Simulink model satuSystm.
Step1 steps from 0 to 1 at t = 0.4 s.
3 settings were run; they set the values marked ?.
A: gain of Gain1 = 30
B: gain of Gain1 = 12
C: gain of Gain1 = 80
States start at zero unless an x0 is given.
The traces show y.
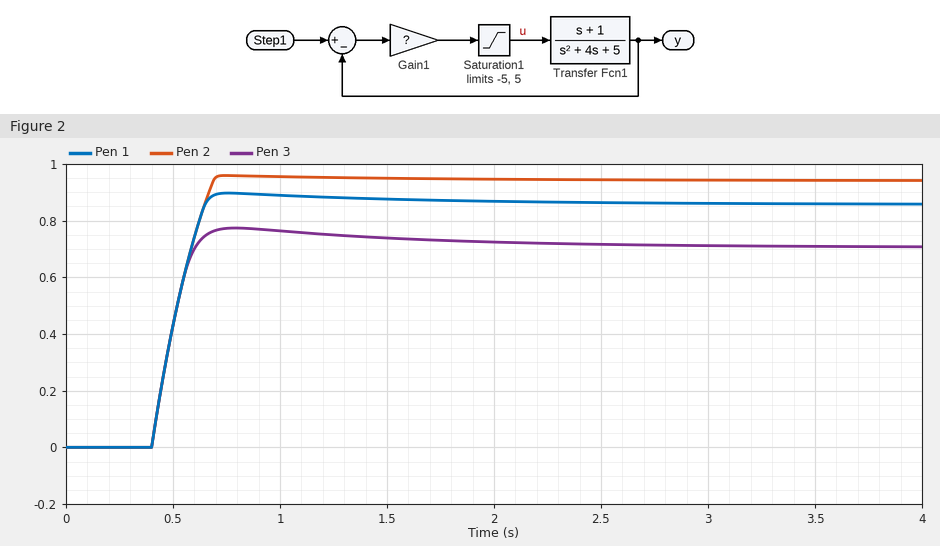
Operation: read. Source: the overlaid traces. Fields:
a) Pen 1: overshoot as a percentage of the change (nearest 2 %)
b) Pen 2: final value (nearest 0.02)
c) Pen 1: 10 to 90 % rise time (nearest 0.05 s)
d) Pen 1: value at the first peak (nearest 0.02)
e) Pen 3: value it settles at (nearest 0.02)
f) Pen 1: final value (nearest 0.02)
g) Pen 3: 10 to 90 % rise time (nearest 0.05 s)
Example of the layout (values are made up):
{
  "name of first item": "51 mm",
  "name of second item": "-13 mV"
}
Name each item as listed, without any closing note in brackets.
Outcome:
{
  "Pen 1: overshoot as a percentage of the change": "4 %",
  "Pen 2: final value": "0.94",
  "Pen 1: 10 to 90 % rise time": "0.20 s",
  "Pen 1: value at the first peak": "0.90",
  "Pen 3: value it settles at": "0.70",
  "Pen 1: final value": "0.86",
  "Pen 3: 10 to 90 % rise time": "0.15 s"
}
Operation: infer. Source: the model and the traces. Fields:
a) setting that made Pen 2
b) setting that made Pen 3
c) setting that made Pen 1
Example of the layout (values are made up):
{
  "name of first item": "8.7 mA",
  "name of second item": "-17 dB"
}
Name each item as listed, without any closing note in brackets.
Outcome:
{
  "setting that made Pen 2": "C",
  "setting that made Pen 3": "B",
  "setting that made Pen 1": "A"
}
